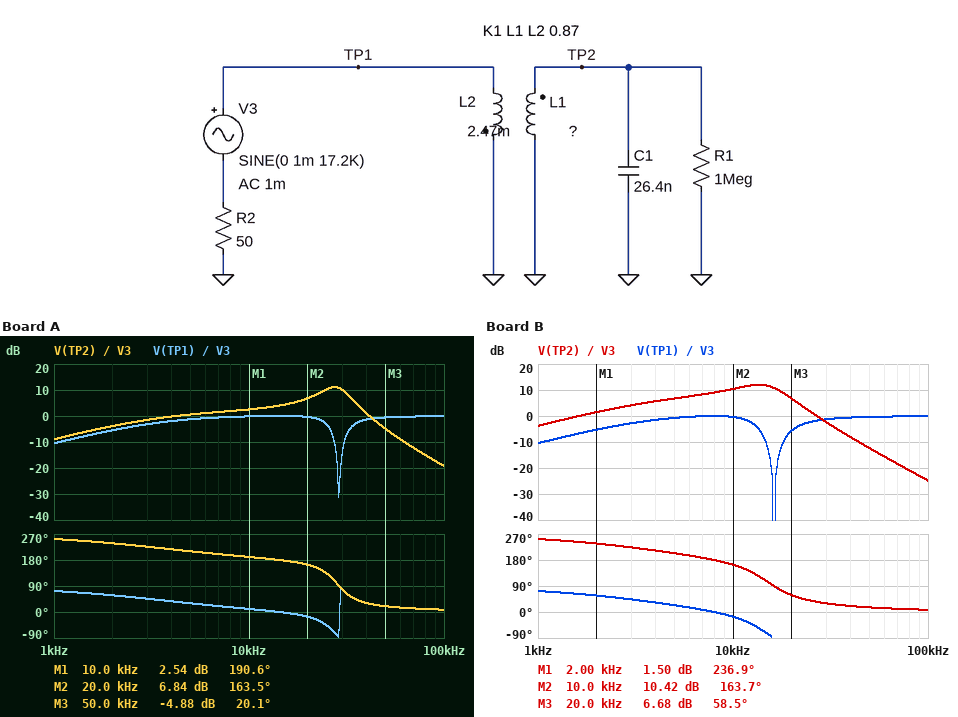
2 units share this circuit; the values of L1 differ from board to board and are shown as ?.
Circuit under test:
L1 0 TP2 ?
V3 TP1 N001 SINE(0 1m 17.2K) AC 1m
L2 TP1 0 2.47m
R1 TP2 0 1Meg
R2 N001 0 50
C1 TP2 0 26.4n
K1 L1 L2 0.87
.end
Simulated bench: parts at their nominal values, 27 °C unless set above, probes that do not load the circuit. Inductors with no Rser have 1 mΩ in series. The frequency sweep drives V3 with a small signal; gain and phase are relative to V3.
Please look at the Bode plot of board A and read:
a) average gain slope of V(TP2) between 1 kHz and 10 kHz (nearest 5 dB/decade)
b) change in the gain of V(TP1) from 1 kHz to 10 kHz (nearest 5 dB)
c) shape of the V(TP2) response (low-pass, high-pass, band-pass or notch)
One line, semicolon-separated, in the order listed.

10 dB/decade; 10 dB; band-pass
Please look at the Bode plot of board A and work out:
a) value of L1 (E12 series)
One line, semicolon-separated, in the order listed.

4.7 mH
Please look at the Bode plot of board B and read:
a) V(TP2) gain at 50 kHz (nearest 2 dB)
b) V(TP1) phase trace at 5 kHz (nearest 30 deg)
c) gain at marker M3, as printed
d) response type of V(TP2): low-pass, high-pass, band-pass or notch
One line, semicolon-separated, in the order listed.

-12 dB; 30 deg; 6.68 dB; band-pass
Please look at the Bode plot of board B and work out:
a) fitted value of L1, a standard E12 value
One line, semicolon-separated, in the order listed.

15 mH
